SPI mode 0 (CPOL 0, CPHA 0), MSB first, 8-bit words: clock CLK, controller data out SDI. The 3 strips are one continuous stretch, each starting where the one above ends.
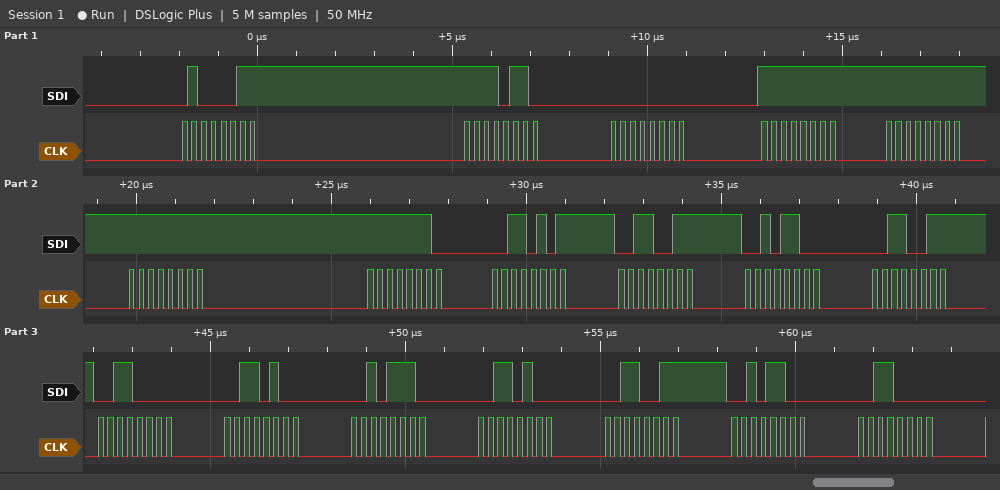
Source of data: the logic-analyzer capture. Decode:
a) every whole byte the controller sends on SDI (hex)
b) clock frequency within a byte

43 F6 00 FF FF FF FE 35 33 2C 33 30 34 2E 34 33 2C 30
4 MHz
